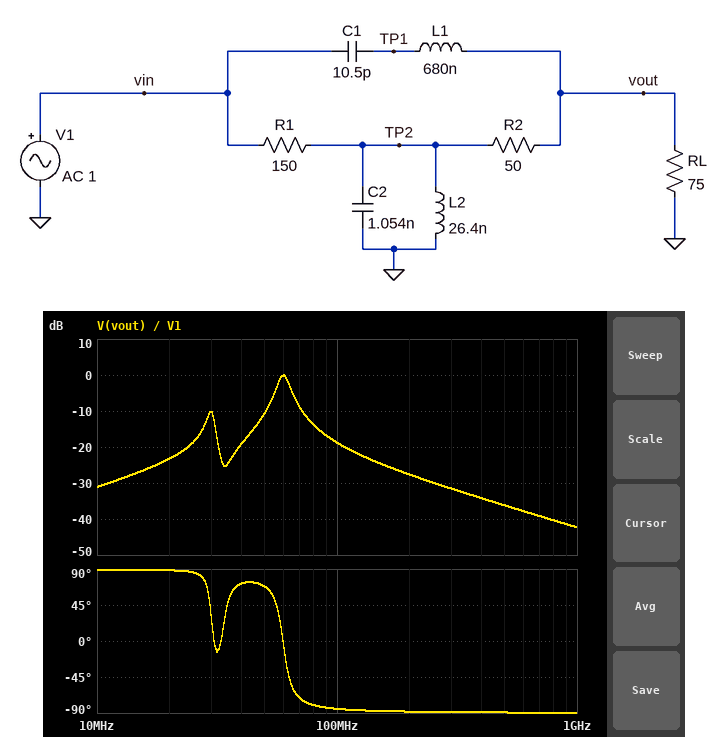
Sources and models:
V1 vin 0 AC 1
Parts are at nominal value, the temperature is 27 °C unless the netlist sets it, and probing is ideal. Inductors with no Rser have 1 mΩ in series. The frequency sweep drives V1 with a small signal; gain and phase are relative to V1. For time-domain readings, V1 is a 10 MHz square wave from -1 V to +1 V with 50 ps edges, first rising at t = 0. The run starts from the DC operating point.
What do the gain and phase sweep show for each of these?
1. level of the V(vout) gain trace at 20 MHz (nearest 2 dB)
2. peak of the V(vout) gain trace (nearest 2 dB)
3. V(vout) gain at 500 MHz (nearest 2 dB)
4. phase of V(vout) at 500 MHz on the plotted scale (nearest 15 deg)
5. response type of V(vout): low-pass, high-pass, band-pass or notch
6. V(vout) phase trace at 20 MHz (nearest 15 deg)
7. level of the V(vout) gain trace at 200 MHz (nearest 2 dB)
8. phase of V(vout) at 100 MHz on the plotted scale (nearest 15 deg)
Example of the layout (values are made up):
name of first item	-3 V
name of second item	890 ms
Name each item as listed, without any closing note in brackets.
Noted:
level of the V(vout) gain trace at 20 MHz	-24 dB
peak of the V(vout) gain trace	0 dB
V(vout) gain at 500 MHz	-36 dB
phase of V(vout) at 500 MHz on the plotted scale	-90 deg
response type of V(vout): low-pass, high-pass, band-pass or notch	band-pass
V(vout) phase trace at 20 MHz	90 deg
level of the V(vout) gain trace at 200 MHz	-28 dB
phase of V(vout) at 100 MHz on the plotted scale	-90 deg
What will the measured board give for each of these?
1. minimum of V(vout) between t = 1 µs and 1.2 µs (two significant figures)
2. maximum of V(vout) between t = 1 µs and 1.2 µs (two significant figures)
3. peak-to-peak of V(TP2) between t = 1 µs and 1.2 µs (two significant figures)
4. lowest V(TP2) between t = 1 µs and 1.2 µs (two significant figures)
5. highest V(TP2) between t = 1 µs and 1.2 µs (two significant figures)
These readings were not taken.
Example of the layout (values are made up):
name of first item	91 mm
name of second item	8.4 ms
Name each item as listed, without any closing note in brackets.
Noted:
minimum of V(vout) between t = 1 µs and 1.2 µs	-280 mV
maximum of V(vout) between t = 1 µs and 1.2 µs	280 mV
peak-to-peak of V(TP2) between t = 1 µs and 1.2 µs	460 mV
lowest V(TP2) between t = 1 µs and 1.2 µs	-230 mV
highest V(TP2) between t = 1 µs and 1.2 µs	230 mV
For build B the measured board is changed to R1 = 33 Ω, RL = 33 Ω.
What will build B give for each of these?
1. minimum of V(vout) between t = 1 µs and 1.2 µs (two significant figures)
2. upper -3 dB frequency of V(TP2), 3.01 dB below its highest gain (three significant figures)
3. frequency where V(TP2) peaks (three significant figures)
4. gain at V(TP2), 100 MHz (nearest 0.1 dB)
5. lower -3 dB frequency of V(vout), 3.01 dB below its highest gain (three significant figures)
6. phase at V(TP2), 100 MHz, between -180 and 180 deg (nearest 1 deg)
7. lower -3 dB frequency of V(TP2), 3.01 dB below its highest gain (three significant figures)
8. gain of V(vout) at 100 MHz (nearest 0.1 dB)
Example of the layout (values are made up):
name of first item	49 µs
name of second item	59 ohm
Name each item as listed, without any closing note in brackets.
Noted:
minimum of V(vout) between t = 1 µs and 1.2 µs	-230 mV
upper -3 dB frequency of V(TP2), 3.01 dB below its highest gain	33.5 MHz
frequency where V(TP2) peaks	30.1 MHz
gain at V(TP2), 100 MHz	-25.9 dB
lower -3 dB frequency of V(vout), 3.01 dB below its highest gain	57.5 MHz
phase at V(TP2), 100 MHz, between -180 and 180 deg	-89 deg
lower -3 dB frequency of V(TP2), 3.01 dB below its highest gain	27.1 MHz
gain of V(vout) at 100 MHz	-20.7 dB
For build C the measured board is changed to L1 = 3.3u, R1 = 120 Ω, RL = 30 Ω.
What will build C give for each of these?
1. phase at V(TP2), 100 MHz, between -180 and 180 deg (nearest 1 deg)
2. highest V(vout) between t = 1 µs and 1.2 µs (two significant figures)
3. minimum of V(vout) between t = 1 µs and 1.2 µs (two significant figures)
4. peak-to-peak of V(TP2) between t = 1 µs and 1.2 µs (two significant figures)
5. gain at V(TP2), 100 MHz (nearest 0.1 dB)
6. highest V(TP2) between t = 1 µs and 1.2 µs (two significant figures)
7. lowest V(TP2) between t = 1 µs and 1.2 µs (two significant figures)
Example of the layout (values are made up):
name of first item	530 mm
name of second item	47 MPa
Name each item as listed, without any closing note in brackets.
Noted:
phase at V(TP2), 100 MHz, between -180 and 180 deg	-89 deg
highest V(vout) between t = 1 µs and 1.2 µs	130 mV
minimum of V(vout) between t = 1 µs and 1.2 µs	-130 mV
peak-to-peak of V(TP2) between t = 1 µs and 1.2 µs	430 mV
gain at V(TP2), 100 MHz	-37.2 dB
highest V(TP2) between t = 1 µs and 1.2 µs	210 mV
lowest V(TP2) between t = 1 µs and 1.2 µs	-210 mV
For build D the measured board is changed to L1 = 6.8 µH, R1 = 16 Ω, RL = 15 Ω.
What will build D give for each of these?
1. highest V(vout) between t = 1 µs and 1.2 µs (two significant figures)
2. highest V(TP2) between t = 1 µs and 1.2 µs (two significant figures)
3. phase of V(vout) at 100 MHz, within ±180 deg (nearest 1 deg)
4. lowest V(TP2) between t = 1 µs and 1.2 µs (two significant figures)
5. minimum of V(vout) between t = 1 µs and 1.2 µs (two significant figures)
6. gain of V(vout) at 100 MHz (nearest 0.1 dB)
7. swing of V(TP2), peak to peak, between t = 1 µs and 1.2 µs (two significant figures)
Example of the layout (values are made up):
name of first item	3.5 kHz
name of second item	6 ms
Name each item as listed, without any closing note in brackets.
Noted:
highest V(vout) between t = 1 µs and 1.2 µs	140 mV
highest V(TP2) between t = 1 µs and 1.2 µs	560 mV
phase of V(vout) at 100 MHz, within ±180 deg	-83 deg
lowest V(TP2) between t = 1 µs and 1.2 µs	-560 mV
minimum of V(vout) between t = 1 µs and 1.2 µs	-150 mV
gain of V(vout) at 100 MHz	-31.5 dB
swing of V(TP2), peak to peak, between t = 1 µs and 1.2 µs	1.1 V
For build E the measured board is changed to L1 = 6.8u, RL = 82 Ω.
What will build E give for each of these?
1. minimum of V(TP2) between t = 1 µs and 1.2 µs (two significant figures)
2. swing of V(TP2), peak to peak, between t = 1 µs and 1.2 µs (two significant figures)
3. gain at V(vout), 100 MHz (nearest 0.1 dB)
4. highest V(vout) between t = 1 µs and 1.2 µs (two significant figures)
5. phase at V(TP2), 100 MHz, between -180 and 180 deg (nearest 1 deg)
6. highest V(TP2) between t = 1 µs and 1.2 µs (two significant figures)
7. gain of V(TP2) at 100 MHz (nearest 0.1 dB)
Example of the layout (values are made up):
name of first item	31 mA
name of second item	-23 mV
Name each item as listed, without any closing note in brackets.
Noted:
minimum of V(TP2) between t = 1 µs and 1.2 µs	-220 mV
swing of V(TP2), peak to peak, between t = 1 µs and 1.2 µs	440 mV
gain at V(vout), 100 MHz	-36.8 dB
highest V(vout) between t = 1 µs and 1.2 µs	170 mV
phase at V(TP2), 100 MHz, between -180 and 180 deg	-90 deg
highest V(TP2) between t = 1 µs and 1.2 µs	220 mV
gain of V(TP2) at 100 MHz	-39.1 dB
